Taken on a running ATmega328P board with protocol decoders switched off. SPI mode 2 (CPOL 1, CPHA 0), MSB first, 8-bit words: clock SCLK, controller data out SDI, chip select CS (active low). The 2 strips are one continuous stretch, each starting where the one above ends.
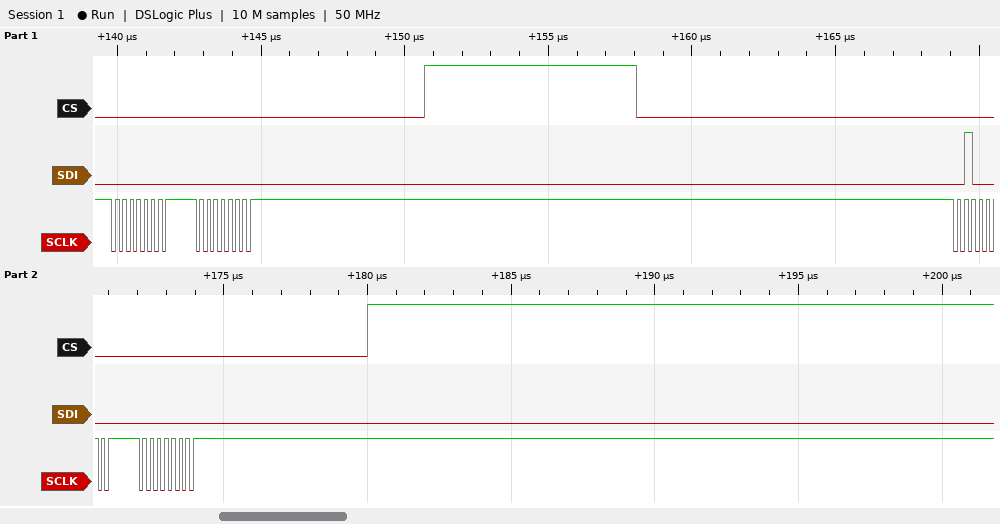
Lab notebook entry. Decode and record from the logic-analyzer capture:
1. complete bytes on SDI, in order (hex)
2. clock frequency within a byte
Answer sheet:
00 00 20 00
4 MHz
